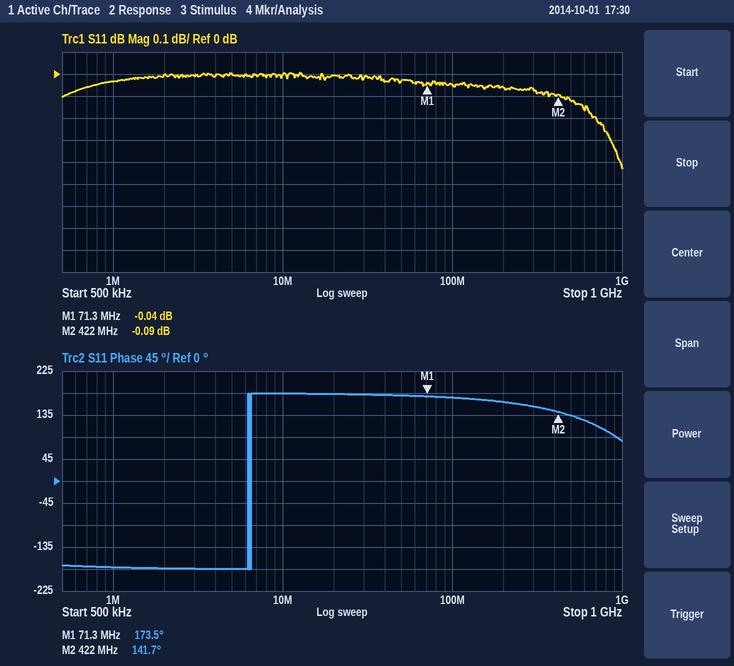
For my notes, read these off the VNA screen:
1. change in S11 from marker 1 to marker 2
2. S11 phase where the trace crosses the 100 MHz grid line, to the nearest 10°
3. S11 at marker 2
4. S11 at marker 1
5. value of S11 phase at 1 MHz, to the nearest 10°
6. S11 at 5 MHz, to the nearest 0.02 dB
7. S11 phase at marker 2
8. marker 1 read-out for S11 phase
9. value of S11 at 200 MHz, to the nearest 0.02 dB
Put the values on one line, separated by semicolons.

-0.05 dB; 170°; -0.09 dB; -0.04 dB; -180°; 0.00 dB; 141.7°; 173.5°; -0.06 dB
